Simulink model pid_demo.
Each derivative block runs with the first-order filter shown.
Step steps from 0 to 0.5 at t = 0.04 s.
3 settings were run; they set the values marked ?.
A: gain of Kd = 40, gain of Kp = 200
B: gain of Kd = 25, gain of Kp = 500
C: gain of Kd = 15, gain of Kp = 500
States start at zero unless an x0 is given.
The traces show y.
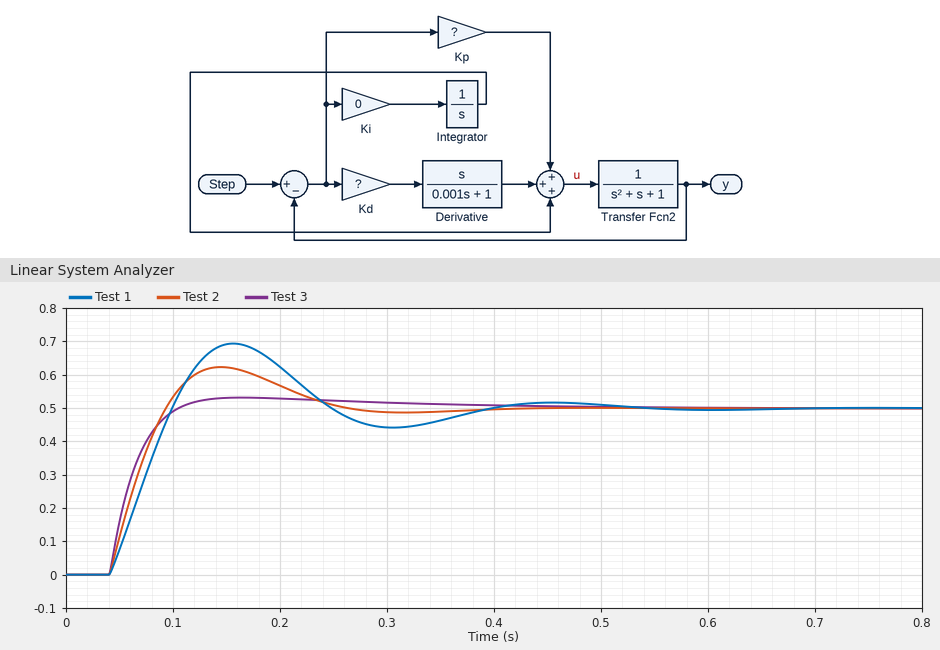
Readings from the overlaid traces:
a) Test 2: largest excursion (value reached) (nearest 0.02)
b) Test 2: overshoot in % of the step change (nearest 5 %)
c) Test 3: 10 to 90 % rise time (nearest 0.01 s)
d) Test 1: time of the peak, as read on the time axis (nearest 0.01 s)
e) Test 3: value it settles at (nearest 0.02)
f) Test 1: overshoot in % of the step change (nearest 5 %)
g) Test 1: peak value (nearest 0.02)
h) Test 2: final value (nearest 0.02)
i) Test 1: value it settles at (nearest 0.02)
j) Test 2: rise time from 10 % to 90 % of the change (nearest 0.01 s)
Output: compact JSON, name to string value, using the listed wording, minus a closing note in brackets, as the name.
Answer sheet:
{"Test 2: largest excursion (value reached)": "0.62", "Test 2: overshoot in % of the step change": "25 %", "Test 3: 10 to 90 % rise time": "0.04 s", "Test 1: time of the peak, as read on the time axis": "0.16 s", "Test 3: value it settles at": "0.50", "Test 1: overshoot in % of the step change": "40 %", "Test 1: peak value": "0.70", "Test 2: final value": "0.50", "Test 1: value it settles at": "0.50", "Test 2: rise time from 10 % to 90 % of the change": "0.04 s"}
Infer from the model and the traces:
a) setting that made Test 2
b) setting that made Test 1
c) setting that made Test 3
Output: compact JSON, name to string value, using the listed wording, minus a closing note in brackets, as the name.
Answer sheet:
{"setting that made Test 2": "B", "setting that made Test 1": "C", "setting that made Test 3": "A"}
